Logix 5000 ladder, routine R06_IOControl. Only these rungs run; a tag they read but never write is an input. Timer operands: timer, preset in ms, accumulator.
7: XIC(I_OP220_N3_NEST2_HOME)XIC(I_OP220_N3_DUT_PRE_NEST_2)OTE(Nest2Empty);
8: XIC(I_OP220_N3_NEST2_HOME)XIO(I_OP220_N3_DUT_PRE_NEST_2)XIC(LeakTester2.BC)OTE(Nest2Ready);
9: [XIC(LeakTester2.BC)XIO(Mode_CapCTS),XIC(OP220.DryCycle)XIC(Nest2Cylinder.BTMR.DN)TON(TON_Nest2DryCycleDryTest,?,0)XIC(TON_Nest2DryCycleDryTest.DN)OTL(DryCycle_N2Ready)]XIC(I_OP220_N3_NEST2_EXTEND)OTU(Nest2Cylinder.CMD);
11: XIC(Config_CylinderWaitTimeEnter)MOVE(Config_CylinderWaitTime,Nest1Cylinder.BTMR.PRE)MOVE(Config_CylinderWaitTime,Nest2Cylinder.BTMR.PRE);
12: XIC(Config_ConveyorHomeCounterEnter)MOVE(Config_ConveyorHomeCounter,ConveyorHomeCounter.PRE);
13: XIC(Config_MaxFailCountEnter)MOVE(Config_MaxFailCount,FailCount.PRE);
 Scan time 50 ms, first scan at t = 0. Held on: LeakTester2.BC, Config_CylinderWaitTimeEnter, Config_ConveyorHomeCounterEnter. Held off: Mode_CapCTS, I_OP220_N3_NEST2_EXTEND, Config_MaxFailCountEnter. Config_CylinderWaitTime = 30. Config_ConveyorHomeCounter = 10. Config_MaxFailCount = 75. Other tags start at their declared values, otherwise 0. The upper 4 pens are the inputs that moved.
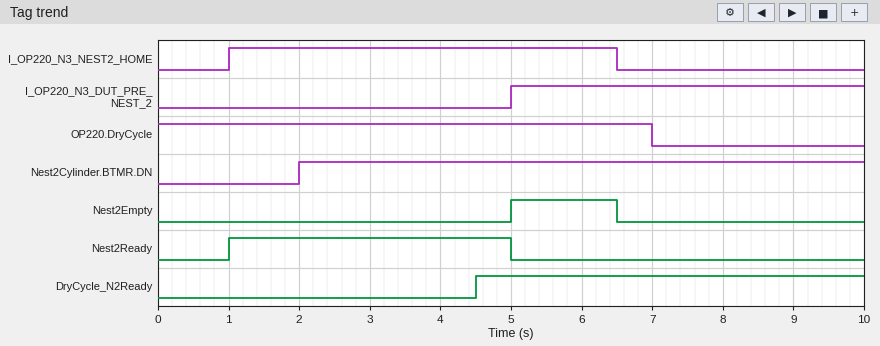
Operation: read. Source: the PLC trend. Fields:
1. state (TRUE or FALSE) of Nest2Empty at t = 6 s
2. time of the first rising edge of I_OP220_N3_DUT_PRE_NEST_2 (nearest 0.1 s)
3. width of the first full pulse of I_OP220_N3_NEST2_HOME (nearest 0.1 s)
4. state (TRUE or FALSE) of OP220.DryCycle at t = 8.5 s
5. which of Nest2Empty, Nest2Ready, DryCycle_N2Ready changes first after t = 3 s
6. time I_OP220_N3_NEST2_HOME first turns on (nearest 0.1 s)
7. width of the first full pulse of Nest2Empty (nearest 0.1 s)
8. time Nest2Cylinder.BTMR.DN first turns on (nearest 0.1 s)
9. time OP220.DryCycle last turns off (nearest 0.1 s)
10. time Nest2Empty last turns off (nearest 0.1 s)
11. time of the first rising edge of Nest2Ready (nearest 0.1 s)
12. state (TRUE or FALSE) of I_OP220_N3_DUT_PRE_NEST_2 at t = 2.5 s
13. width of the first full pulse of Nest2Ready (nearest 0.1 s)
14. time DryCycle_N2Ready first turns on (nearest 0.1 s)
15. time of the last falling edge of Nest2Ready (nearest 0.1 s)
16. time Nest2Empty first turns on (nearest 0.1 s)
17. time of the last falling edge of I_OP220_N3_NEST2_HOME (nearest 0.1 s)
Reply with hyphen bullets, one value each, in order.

- TRUE
- 5.0 s
- 5.5 s
- FALSE
- DryCycle_N2Ready
- 1.0 s
- 1.5 s
- 2.0 s
- 7.0 s
- 6.5 s
- 1.0 s
- FALSE
- 4.0 s
- 4.5 s
- 5.0 s
- 5.0 s
- 6.5 s
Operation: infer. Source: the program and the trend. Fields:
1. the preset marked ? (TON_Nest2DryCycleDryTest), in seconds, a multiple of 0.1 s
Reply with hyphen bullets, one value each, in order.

- 2.5 s
